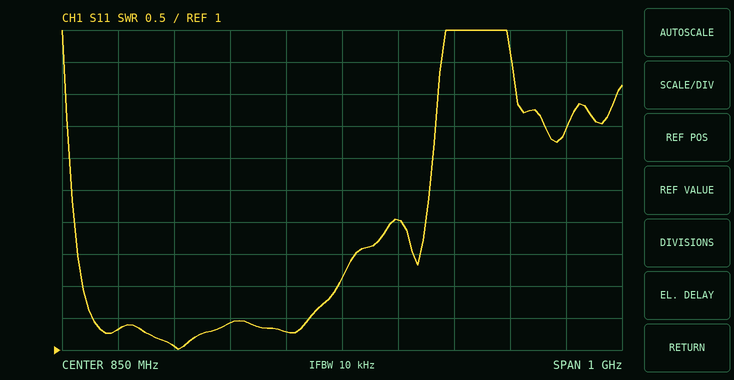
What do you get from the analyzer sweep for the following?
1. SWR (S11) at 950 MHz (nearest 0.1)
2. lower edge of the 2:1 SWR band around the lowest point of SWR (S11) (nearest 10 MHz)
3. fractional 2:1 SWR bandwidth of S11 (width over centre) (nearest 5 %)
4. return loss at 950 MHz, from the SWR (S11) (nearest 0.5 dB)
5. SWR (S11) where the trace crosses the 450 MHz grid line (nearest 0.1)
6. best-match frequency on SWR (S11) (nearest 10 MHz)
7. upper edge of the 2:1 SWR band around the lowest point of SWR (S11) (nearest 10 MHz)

3.0
390 MHz
75 %
6.0 dB
1.3
560 MHz
840 MHz
